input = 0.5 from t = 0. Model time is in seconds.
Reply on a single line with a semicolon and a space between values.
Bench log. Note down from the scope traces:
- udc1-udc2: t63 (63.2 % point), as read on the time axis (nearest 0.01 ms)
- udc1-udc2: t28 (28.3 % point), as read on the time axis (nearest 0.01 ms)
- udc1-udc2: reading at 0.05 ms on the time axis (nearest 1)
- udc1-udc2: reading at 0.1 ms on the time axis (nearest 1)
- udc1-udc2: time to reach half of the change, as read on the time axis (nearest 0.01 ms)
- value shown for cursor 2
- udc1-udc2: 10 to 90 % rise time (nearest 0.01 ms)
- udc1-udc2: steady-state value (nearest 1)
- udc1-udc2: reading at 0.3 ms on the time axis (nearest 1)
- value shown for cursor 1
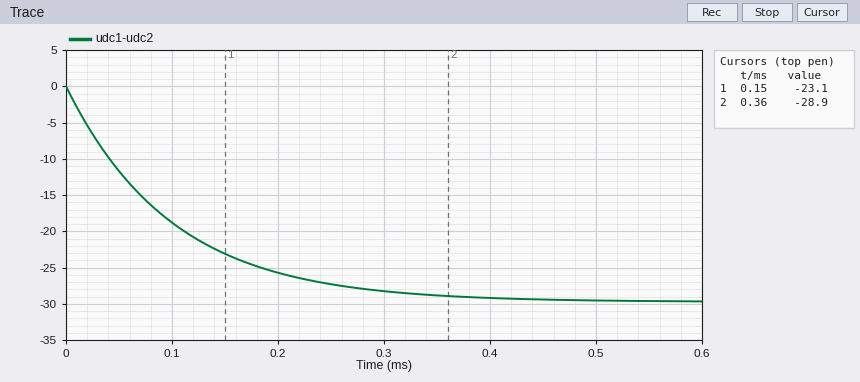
0.10 ms; 0.03 ms; -12; -19; 0.07 ms; -28.9; 0.22 ms; -30; -28; -23.1
